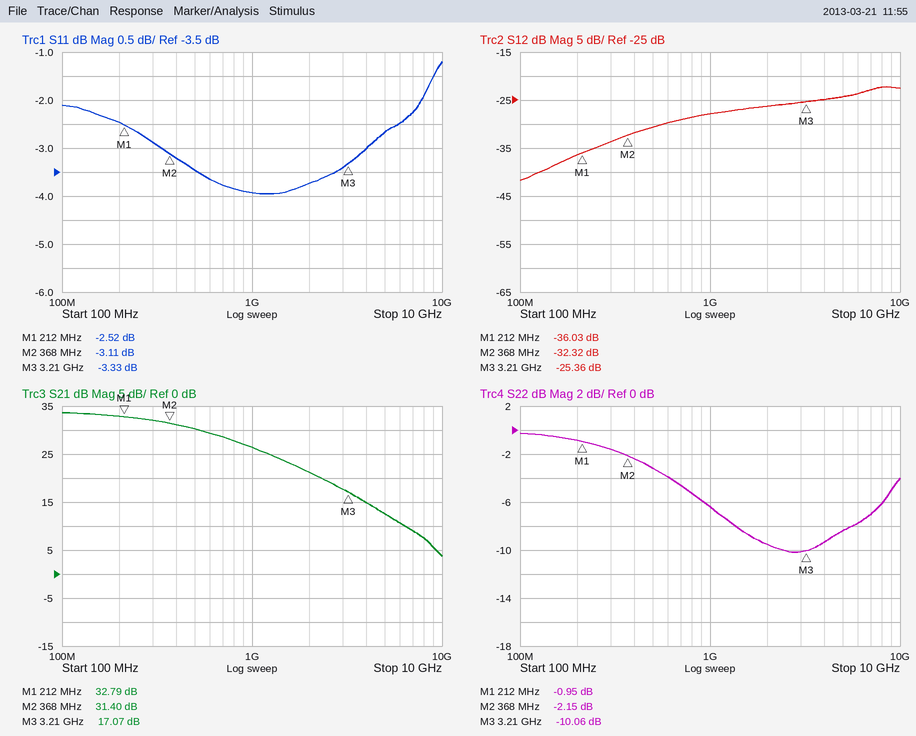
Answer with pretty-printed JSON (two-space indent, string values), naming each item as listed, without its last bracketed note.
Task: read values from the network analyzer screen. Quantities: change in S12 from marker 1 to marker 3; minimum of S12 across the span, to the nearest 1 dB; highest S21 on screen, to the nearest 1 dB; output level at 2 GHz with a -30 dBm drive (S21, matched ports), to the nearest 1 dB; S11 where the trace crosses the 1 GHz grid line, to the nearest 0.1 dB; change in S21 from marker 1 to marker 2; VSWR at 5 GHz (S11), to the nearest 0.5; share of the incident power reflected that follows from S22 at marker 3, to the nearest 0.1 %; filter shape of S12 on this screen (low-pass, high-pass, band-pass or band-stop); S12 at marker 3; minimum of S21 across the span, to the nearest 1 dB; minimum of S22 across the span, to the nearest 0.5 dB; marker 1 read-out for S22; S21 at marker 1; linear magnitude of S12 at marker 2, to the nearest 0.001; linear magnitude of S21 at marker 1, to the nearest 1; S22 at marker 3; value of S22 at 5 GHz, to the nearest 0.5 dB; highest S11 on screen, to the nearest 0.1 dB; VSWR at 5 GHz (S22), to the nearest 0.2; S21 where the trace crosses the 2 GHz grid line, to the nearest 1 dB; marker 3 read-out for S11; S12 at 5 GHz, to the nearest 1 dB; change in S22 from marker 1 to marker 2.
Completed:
{
  "change in S12 from marker 1 to marker 3": "10.67 dB",
  "minimum of S12 across the span, to the nearest 1 dB": "-42 dB",
  "highest S21 on screen, to the nearest 1 dB": "34 dB",
  "output level at 2 GHz with a -30 dBm drive (S21, matched ports), to the nearest 1 dB": "-9 dBm",
  "S11 where the trace crosses the 1 GHz grid line, to the nearest 0.1 dB": "-3.9 dB",
  "change in S21 from marker 1 to marker 2": "-1.39 dB",
  "VSWR at 5 GHz (S11), to the nearest 0.5": "6.5",
  "share of the incident power reflected that follows from S22 at marker 3, to the nearest 0.1 %": "9.9 %",
  "filter shape of S12 on this screen": "high-pass",
  "S12 at marker 3": "-25.36 dB",
  "minimum of S21 across the span, to the nearest 1 dB": "4 dB",
  "minimum of S22 across the span, to the nearest 0.5 dB": "-10.0 dB",
  "marker 1 read-out for S22": "-0.95 dB",
  "S21 at marker 1": "32.79 dB",
  "linear magnitude of S12 at marker 2, to the nearest 0.001": "0.024",
  "linear magnitude of S21 at marker 1, to the nearest 1": "44",
  "S22 at marker 3": "-10.06 dB",
  "value of S22 at 5 GHz, to the nearest 0.5 dB": "-8.5 dB",
  "highest S11 on screen, to the nearest 0.1 dB": "-1.2 dB",
  "VSWR at 5 GHz (S22), to the nearest 0.2": "2.2",
  "S21 where the trace crosses the 2 GHz grid line, to the nearest 1 dB": "21 dB",
  "marker 3 read-out for S11": "-3.33 dB",
  "S12 at 5 GHz, to the nearest 1 dB": "-24 dB",
  "change in S22 from marker 1 to marker 2": "-1.20 dB"
}
